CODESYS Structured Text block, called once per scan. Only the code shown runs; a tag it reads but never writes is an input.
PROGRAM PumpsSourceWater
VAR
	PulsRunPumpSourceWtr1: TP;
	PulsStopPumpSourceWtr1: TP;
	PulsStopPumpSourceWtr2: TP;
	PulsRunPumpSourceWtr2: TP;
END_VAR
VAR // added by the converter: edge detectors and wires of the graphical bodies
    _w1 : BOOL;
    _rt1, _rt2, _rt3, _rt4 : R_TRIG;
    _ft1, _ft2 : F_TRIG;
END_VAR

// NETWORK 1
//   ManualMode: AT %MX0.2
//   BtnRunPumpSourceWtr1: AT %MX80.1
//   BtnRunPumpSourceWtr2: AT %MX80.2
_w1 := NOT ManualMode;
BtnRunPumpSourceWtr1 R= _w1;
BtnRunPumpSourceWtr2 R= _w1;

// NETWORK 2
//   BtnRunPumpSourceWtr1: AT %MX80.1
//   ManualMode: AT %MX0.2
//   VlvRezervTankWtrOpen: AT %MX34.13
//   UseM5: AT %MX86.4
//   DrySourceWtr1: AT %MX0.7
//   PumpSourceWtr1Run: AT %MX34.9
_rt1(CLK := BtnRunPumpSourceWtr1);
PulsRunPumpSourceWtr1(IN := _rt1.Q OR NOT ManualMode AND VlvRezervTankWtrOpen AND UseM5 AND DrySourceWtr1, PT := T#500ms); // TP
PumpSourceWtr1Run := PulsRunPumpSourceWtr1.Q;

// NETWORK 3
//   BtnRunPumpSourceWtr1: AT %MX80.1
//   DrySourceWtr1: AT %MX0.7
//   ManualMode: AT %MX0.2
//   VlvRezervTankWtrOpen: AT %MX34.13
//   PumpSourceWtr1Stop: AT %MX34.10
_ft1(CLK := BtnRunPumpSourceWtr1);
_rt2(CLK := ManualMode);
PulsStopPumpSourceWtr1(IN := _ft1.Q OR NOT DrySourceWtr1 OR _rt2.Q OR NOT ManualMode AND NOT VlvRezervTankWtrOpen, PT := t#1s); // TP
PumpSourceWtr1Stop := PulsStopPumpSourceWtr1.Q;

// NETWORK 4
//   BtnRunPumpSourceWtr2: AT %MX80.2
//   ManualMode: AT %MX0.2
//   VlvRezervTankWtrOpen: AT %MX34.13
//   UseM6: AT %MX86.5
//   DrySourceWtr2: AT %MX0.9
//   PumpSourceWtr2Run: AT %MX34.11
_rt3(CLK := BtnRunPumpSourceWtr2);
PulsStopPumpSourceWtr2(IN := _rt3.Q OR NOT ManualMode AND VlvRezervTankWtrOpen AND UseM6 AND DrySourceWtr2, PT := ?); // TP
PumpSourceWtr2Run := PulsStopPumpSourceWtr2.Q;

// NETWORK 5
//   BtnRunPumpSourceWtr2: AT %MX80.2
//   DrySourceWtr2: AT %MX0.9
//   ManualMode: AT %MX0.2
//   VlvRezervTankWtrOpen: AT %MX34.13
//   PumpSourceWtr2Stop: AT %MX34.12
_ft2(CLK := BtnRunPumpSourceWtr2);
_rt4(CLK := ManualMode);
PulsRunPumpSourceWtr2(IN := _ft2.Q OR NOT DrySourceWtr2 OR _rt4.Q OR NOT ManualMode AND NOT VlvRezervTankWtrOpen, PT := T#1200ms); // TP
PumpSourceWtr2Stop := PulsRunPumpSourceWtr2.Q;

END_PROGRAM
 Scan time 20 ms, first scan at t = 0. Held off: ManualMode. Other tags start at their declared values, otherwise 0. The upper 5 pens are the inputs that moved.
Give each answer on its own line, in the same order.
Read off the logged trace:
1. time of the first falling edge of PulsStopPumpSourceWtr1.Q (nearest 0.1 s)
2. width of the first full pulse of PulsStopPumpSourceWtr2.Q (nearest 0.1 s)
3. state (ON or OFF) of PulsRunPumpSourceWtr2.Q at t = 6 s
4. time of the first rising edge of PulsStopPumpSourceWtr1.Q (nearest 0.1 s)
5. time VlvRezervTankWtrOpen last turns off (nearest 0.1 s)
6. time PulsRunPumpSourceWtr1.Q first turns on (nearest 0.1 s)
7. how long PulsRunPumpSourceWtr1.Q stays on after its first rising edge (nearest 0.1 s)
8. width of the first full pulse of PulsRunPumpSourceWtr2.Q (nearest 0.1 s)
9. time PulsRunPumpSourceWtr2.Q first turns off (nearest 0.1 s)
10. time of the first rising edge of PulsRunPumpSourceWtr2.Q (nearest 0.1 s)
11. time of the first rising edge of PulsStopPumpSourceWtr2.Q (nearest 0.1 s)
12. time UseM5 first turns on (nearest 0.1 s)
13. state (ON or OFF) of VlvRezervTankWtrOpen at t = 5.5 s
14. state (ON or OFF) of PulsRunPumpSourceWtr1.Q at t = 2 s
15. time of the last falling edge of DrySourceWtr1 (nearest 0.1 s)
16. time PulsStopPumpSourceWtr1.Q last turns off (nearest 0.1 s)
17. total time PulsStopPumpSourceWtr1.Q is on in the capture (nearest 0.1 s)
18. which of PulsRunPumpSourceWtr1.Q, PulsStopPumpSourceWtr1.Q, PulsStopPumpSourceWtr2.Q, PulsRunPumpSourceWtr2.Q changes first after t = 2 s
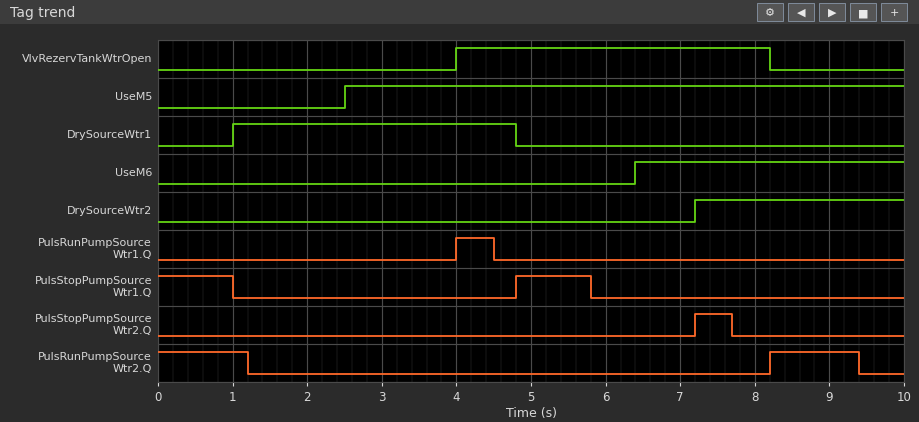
1.0 s
0.5 s
OFF
4.8 s
8.2 s
4.0 s
0.5 s
1.2 s
1.2 s
8.2 s
7.2 s
2.5 s
ON
OFF
4.8 s
5.8 s
2.0 s
PulsRunPumpSourceWtr1.Q
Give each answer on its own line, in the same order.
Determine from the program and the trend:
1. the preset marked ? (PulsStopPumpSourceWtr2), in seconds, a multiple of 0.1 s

0.5 s
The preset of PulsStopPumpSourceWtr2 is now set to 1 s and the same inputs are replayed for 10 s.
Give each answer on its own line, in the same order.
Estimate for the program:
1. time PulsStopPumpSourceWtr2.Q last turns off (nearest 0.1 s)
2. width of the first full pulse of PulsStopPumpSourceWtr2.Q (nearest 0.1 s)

8.2 s
1.0 s
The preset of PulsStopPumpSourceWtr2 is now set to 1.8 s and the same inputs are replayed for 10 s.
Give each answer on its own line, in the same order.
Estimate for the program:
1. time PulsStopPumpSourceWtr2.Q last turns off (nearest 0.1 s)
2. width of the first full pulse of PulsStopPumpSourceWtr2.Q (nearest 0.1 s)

9.0 s
1.8 s
